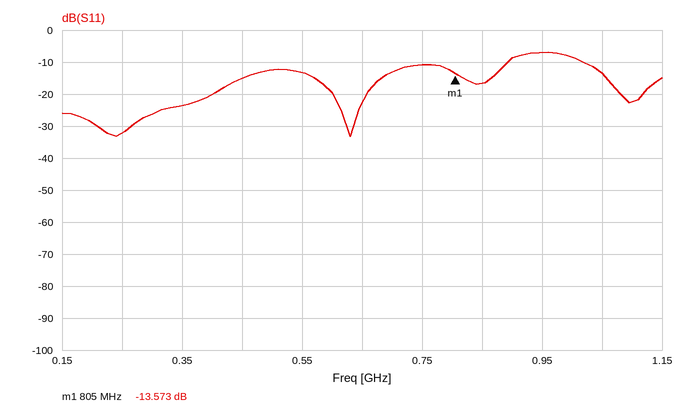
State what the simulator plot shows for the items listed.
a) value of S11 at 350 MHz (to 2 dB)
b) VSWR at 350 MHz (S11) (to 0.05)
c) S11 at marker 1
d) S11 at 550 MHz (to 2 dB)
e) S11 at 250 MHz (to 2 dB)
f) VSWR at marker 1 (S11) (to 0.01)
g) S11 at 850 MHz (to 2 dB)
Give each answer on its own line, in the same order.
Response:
-24 dB
1.15
-13.573 dB
-14 dB
-32 dB
1.53
-16 dB
